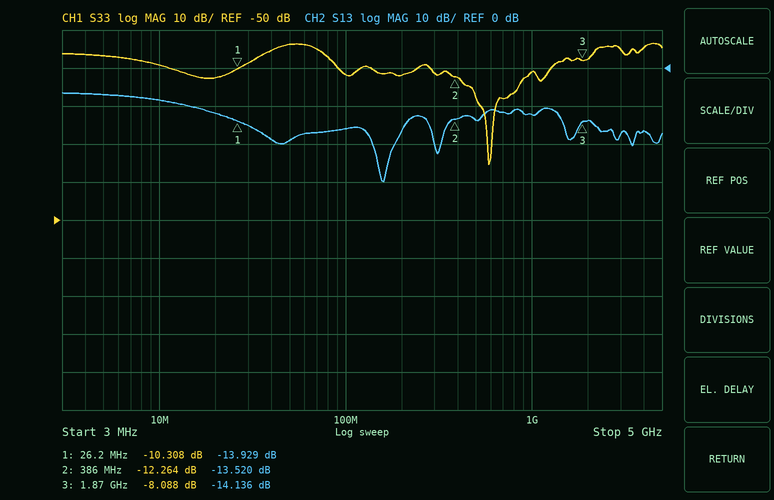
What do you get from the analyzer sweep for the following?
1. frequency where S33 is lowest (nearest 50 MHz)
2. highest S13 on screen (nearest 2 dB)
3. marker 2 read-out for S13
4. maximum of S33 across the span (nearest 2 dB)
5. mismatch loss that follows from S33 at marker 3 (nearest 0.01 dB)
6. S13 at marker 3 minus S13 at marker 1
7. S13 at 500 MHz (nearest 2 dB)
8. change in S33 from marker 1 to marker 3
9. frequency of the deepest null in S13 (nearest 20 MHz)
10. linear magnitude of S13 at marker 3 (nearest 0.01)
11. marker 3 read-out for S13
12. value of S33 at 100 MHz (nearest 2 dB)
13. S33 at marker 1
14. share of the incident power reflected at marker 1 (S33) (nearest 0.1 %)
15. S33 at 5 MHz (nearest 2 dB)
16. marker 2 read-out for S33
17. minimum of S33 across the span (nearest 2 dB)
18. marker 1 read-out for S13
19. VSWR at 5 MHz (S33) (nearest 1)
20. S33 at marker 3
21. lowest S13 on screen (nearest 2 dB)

600 MHz
-6 dB
-13.520 dB
-4 dB
0.73 dB
-0.207 dB
-14 dB
2.220 dB
160 MHz
0.20
-14.136 dB
-12 dB
-10.308 dB
9.3 %
-6 dB
-12.264 dB
-36 dB
-13.929 dB
3
-8.088 dB
-30 dB
